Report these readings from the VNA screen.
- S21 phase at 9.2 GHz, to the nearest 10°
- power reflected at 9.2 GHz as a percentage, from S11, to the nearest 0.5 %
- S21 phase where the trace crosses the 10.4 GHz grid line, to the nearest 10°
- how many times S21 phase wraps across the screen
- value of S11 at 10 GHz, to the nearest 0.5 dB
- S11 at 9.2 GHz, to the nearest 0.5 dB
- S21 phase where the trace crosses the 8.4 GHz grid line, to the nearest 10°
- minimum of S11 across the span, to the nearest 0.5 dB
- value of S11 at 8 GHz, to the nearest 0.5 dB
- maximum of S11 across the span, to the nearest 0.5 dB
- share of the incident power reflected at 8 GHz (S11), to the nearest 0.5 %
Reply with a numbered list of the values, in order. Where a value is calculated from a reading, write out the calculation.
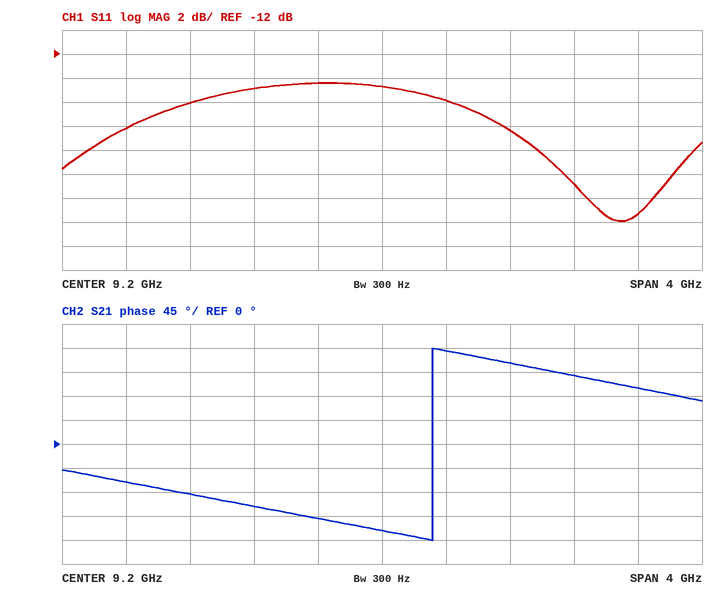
1. -160°
2. 10^(-14.5/10) ≈ 3.5 %
3. 130°
4. 1
5. -18.5 dB
6. -14.5 dB
7. -120°
8. -26.0 dB
9. -16.0 dB
10. -14.5 dB
11. 10^(-16/10) ≈ 2.5 %
